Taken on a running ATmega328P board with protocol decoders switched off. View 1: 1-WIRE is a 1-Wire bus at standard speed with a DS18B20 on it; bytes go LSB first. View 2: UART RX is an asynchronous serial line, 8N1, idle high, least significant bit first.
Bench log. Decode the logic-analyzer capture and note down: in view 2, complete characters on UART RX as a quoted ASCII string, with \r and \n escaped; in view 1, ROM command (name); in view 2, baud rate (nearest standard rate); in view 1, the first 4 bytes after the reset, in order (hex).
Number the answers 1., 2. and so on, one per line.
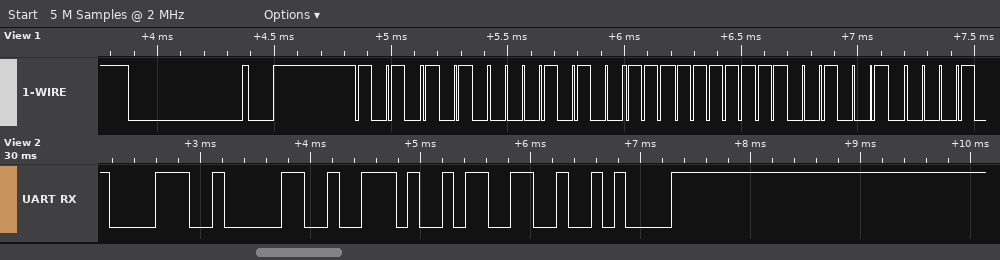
1. "80.3\n"
2. Match ROM
3. 9600 baud
4. 55 28 FF 93
